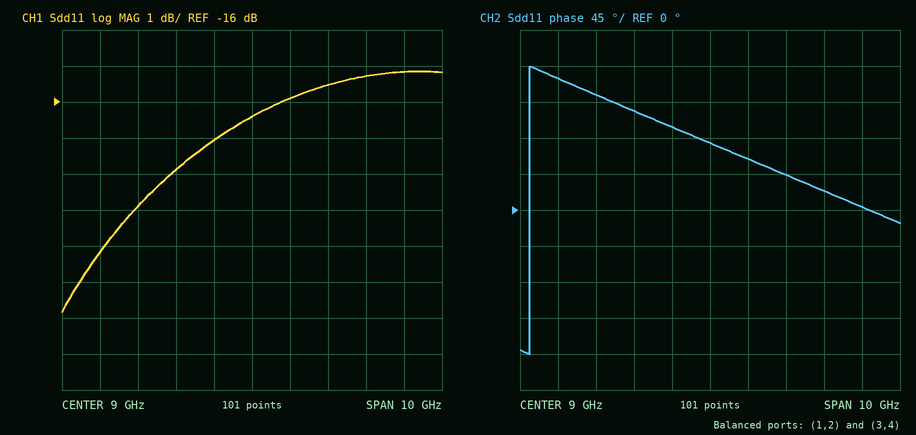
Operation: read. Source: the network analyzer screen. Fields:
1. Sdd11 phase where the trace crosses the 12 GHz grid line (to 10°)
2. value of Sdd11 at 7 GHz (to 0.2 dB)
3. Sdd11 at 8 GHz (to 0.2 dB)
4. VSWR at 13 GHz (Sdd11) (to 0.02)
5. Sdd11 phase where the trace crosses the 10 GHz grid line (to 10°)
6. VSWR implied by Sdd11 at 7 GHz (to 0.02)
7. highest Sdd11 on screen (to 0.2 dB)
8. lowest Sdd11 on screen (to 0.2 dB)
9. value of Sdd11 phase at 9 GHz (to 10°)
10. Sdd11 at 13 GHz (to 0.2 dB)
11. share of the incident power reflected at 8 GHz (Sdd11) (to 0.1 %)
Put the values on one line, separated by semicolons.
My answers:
20°; -17.8 dB; -17.0 dB; 1.42; 60°; 1.30; -15.2 dB; -21.8 dB; 80°; -15.2 dB; 2.0 %
